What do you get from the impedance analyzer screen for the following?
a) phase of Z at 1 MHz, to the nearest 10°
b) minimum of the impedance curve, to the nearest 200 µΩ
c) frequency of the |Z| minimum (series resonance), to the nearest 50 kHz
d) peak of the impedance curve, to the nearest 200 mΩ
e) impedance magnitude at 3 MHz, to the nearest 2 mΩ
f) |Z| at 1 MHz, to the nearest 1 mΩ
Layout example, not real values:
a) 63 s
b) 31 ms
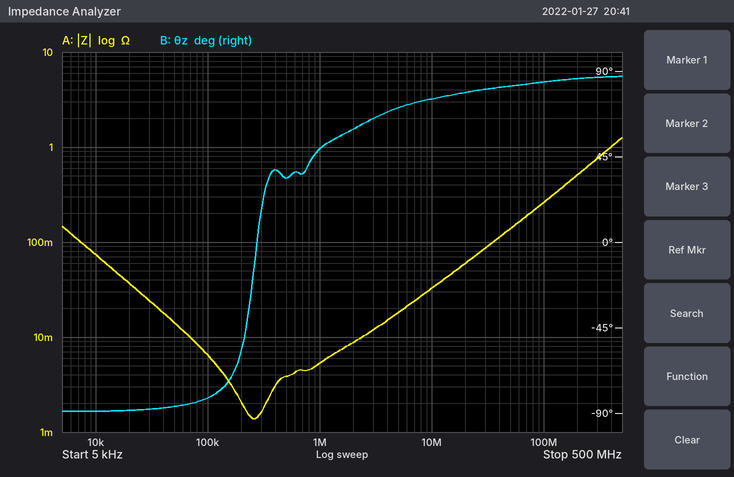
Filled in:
a) 50°
b) 1.4 mΩ
c) 250 kHz
d) 1.2 Ω
e) 12 mΩ
f) 5 mΩ
